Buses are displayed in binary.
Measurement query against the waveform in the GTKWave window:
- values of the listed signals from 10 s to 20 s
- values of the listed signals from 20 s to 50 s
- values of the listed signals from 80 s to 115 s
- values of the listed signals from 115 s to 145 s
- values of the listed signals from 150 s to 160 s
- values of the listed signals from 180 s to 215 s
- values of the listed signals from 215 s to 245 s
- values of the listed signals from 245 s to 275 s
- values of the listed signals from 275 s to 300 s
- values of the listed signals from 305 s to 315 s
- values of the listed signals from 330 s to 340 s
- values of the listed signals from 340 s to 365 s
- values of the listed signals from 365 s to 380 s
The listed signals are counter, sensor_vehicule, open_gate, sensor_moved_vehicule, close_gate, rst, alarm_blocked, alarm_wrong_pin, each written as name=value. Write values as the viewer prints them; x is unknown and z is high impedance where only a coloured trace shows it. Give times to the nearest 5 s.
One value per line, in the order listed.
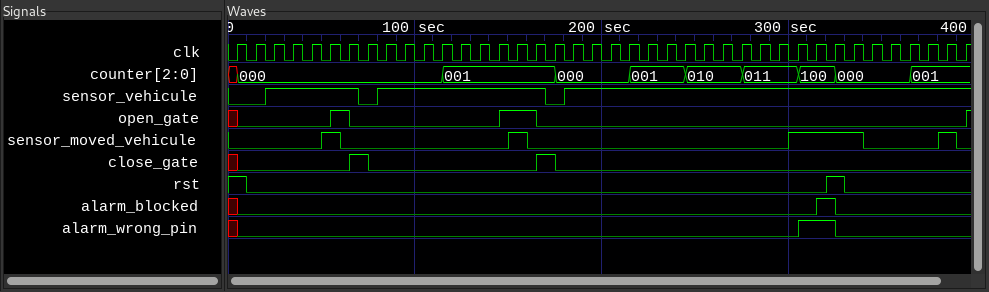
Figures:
counter=000, sensor_vehicule=0, open_gate=0, sensor_moved_vehicule=0, close_gate=0, rst=0, alarm_blocked=0, alarm_wrong_pin=0
counter=000, sensor_vehicule=1, open_gate=0, sensor_moved_vehicule=0, close_gate=0, rst=0, alarm_blocked=0, alarm_wrong_pin=0
counter=000, sensor_vehicule=1, open_gate=0, sensor_moved_vehicule=0, close_gate=0, rst=0, alarm_blocked=0, alarm_wrong_pin=0
counter=001, sensor_vehicule=1, open_gate=0, sensor_moved_vehicule=0, close_gate=0, rst=0, alarm_blocked=0, alarm_wrong_pin=0
counter=001, sensor_vehicule=1, open_gate=1, sensor_moved_vehicule=1, close_gate=0, rst=0, alarm_blocked=0, alarm_wrong_pin=0
counter=000, sensor_vehicule=1, open_gate=0, sensor_moved_vehicule=0, close_gate=0, rst=0, alarm_blocked=0, alarm_wrong_pin=0
counter=001, sensor_vehicule=1, open_gate=0, sensor_moved_vehicule=0, close_gate=0, rst=0, alarm_blocked=0, alarm_wrong_pin=0
counter=010, sensor_vehicule=1, open_gate=0, sensor_moved_vehicule=0, close_gate=0, rst=0, alarm_blocked=0, alarm_wrong_pin=0
counter=011, sensor_vehicule=1, open_gate=0, sensor_moved_vehicule=0, close_gate=0, rst=0, alarm_blocked=0, alarm_wrong_pin=0
counter=100, sensor_vehicule=1, open_gate=0, sensor_moved_vehicule=1, close_gate=0, rst=0, alarm_blocked=0, alarm_wrong_pin=1
counter=000, sensor_vehicule=1, open_gate=0, sensor_moved_vehicule=1, close_gate=0, rst=0, alarm_blocked=0, alarm_wrong_pin=0
counter=000, sensor_vehicule=1, open_gate=0, sensor_moved_vehicule=0, close_gate=0, rst=0, alarm_blocked=0, alarm_wrong_pin=0
counter=001, sensor_vehicule=1, open_gate=0, sensor_moved_vehicule=0, close_gate=0, rst=0, alarm_blocked=0, alarm_wrong_pin=0
